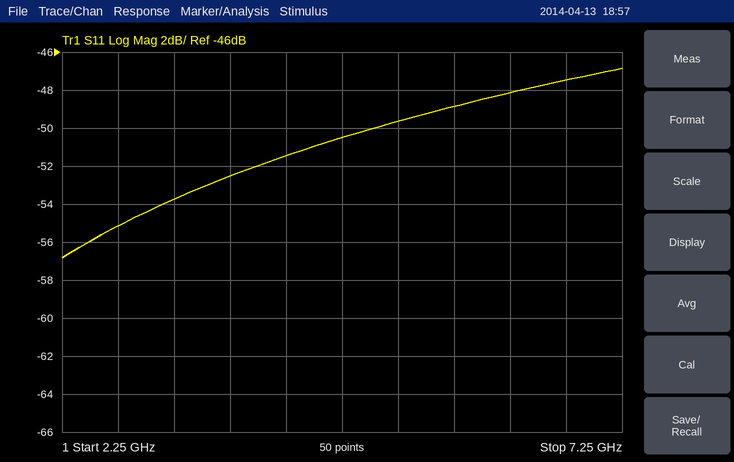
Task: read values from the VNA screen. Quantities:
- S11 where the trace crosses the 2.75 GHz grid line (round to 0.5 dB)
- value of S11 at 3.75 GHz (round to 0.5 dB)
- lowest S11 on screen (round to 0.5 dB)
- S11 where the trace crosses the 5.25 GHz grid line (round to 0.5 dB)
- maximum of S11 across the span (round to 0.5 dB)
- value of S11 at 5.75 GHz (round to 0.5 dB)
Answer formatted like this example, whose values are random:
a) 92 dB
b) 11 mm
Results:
a) -55.0 dB
b) -52.5 dB
c) -57.0 dB
d) -49.5 dB
e) -47.0 dB
f) -49.0 dB
